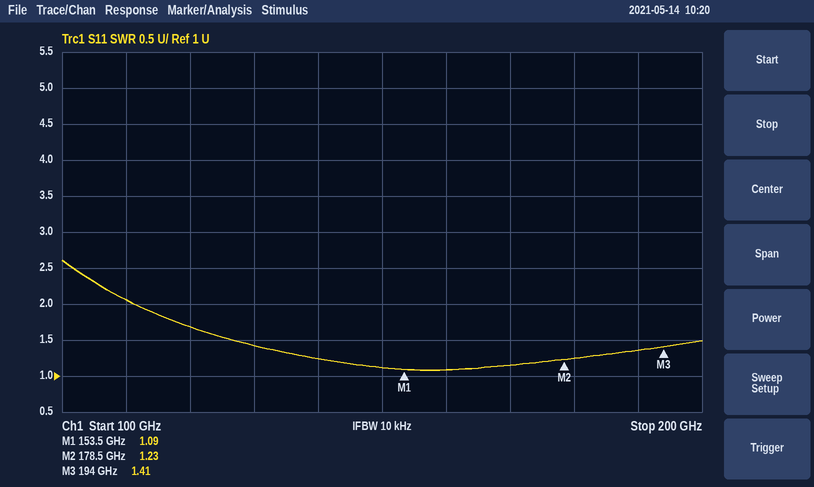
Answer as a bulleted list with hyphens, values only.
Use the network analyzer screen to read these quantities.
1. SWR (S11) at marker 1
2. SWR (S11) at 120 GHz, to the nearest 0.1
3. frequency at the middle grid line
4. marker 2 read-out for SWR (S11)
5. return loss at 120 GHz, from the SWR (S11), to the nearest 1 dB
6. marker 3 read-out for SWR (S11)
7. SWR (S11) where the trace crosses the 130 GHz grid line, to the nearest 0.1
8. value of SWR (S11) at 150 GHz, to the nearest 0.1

- 1.09
- 1.7
- 150 GHz
- 1.23
- 12 dB
- 1.41
- 1.4
- 1.1
